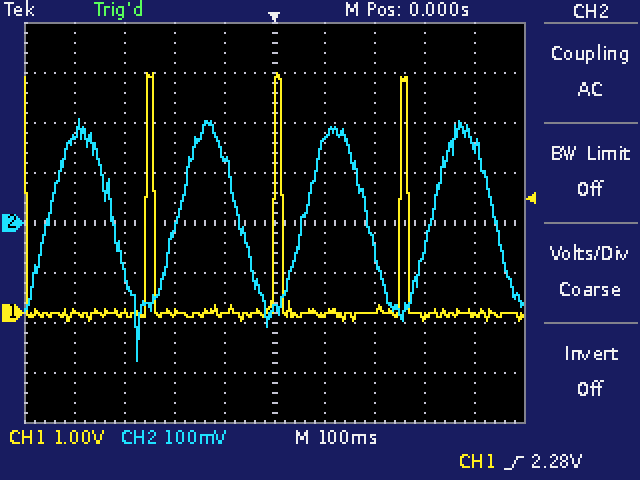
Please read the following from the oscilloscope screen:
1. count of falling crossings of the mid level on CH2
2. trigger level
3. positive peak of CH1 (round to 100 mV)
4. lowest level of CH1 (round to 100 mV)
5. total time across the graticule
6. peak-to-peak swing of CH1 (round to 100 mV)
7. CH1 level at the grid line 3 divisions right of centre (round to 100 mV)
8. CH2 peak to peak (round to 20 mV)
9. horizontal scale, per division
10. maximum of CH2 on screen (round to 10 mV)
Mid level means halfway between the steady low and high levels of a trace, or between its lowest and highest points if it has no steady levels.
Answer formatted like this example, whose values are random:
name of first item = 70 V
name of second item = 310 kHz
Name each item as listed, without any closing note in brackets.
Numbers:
count of falling crossings of the mid level on CH2 = 4
trigger level = 2.28 V
positive peak of CH1 = 4.8 V
lowest level of CH1 = -200 mV
total time across the graticule = 1 s
peak-to-peak swing of CH1 = 5.0 V
CH1 level at the grid line 3 divisions right of centre = -100 mV
CH2 peak to peak = 480 mV
horizontal scale, per division = 100 ms
maximum of CH2 on screen = 210 mV
